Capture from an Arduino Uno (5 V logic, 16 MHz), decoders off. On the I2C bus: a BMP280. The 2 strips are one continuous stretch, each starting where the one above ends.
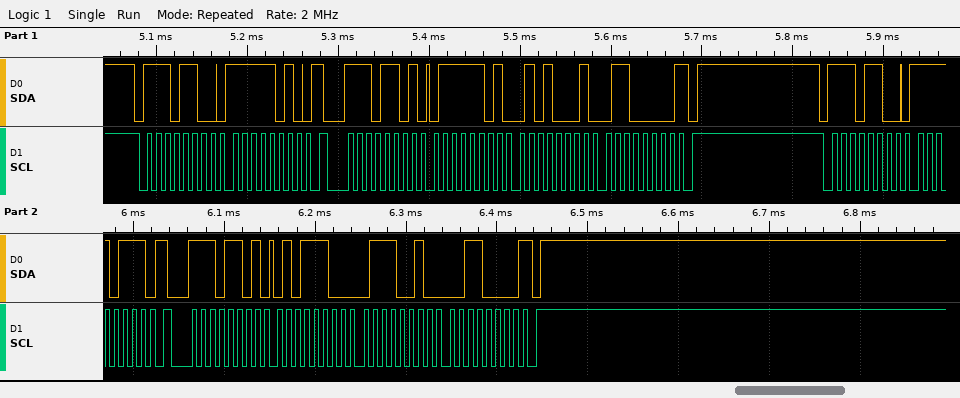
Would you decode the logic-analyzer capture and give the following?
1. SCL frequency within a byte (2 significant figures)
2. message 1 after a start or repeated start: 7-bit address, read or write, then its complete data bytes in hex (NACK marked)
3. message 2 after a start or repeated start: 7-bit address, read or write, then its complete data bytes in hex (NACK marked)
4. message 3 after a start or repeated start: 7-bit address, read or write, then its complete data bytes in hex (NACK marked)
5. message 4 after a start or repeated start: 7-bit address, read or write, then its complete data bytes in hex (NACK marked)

100 kHz
0x76 write: FA
0x76 read: 7D 51 60 NACK
0x76 write: F7
0x76 read: 5C 72 30 NACK
